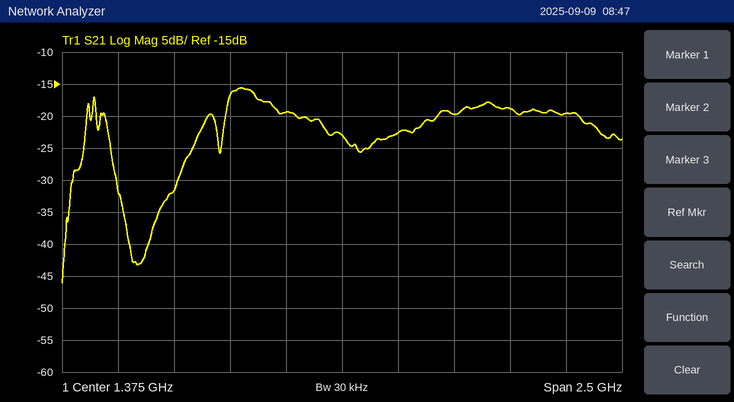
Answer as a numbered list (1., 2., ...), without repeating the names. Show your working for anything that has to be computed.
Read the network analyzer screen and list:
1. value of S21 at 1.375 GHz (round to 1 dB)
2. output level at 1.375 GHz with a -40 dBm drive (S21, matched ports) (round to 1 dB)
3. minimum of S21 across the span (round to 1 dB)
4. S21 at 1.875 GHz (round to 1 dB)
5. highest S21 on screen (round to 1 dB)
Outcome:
1. -23 dB
2. -40 dBm + (-23 dB) = -63 dBm
3. -46 dB
4. -20 dB
5. -16 dB
